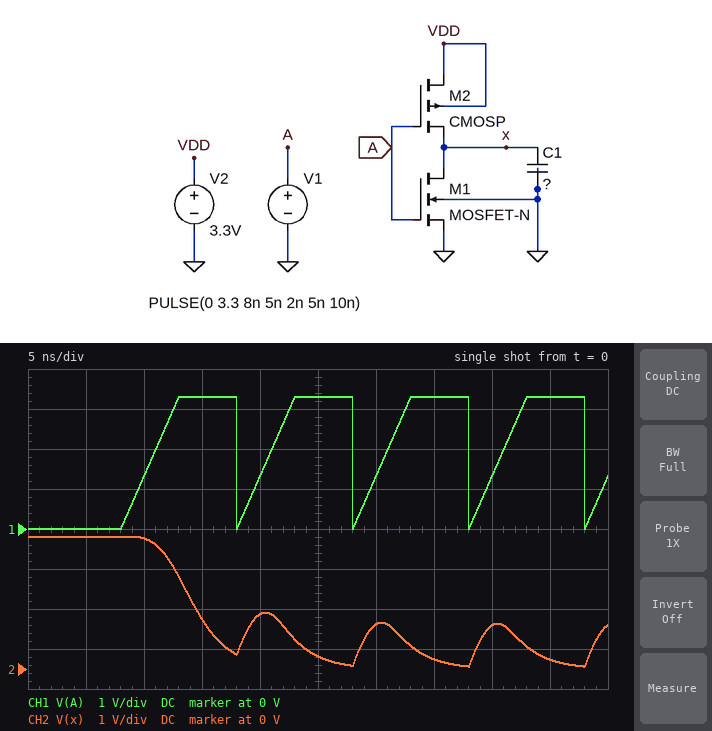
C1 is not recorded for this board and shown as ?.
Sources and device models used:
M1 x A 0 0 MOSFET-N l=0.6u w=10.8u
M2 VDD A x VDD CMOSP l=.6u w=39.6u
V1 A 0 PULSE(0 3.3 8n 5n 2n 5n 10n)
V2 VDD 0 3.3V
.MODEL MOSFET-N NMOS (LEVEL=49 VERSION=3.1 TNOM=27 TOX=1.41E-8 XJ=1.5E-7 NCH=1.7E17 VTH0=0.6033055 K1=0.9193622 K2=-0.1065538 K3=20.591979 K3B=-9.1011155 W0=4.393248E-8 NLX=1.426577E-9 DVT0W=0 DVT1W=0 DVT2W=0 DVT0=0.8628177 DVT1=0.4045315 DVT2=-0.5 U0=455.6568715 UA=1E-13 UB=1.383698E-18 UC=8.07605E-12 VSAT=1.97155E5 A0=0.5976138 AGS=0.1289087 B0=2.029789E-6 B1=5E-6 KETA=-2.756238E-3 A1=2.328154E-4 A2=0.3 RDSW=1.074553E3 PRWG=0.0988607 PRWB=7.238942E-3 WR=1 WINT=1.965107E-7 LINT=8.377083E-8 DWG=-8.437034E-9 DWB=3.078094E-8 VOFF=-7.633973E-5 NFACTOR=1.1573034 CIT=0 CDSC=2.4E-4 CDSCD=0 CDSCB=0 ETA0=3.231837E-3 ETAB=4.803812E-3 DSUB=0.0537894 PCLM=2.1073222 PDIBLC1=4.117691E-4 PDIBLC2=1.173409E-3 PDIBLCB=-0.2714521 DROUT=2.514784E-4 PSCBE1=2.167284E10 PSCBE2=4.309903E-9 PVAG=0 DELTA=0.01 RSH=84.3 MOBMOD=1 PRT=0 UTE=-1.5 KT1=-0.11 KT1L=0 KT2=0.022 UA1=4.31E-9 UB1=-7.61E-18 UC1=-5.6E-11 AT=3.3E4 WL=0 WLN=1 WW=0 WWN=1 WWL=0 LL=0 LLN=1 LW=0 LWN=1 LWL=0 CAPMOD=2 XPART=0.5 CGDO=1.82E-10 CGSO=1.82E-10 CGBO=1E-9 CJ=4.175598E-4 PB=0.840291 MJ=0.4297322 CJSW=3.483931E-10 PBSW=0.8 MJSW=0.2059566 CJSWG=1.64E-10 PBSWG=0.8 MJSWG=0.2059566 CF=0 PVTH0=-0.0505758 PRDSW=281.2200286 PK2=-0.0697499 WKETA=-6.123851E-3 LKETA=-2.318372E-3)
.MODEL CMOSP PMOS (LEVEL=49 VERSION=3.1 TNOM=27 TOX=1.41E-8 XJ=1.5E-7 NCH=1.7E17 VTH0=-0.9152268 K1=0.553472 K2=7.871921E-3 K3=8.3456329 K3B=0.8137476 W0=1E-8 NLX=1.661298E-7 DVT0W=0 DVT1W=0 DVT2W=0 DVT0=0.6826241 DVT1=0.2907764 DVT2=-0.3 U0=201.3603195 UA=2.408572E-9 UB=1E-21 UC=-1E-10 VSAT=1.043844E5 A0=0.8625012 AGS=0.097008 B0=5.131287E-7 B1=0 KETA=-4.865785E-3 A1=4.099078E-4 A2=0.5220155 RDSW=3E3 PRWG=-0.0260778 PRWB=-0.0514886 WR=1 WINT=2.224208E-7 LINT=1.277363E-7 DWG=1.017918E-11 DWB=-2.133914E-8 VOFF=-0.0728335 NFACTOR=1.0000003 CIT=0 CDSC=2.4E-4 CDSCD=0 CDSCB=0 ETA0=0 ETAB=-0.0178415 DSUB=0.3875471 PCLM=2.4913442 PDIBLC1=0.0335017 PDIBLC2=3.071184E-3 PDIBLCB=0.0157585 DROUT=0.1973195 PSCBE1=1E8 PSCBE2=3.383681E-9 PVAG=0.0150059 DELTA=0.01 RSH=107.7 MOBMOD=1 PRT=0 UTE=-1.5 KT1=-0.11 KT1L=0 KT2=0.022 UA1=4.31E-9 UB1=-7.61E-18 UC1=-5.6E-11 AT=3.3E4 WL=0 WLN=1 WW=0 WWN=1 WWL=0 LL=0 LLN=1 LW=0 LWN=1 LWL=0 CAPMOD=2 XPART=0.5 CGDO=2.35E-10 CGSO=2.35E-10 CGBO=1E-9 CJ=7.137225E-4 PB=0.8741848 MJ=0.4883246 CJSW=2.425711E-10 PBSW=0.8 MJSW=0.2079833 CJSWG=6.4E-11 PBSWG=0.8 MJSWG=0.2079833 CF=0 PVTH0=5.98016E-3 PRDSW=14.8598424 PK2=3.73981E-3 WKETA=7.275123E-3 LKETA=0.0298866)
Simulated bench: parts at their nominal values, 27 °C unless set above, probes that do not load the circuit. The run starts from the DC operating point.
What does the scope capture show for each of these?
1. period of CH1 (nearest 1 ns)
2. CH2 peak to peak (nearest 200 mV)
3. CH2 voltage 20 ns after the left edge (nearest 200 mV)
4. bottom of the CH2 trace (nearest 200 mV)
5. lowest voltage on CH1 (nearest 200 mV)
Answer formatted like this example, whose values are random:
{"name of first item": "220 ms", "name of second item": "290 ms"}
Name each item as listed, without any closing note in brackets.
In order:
{"period of CH1": "10 ns", "CH2 peak to peak": "3.2 V", "CH2 voltage 20 ns after the left edge": "1.4 V", "bottom of the CH2 trace": "0 V", "lowest voltage on CH1": "0 V"}
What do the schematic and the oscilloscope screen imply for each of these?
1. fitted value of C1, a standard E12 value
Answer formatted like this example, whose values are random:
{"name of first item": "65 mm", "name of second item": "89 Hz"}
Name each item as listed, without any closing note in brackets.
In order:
{"fitted value of C1, a standard E12 value": "4.7 pF"}
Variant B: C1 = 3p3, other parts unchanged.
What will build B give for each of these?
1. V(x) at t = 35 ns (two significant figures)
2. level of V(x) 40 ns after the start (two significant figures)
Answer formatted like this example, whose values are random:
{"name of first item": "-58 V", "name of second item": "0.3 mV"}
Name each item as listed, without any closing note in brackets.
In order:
{"V(x) at t = 35 ns": "170 mV", "level of V(x) 40 ns after the start": "1.5 V"}
